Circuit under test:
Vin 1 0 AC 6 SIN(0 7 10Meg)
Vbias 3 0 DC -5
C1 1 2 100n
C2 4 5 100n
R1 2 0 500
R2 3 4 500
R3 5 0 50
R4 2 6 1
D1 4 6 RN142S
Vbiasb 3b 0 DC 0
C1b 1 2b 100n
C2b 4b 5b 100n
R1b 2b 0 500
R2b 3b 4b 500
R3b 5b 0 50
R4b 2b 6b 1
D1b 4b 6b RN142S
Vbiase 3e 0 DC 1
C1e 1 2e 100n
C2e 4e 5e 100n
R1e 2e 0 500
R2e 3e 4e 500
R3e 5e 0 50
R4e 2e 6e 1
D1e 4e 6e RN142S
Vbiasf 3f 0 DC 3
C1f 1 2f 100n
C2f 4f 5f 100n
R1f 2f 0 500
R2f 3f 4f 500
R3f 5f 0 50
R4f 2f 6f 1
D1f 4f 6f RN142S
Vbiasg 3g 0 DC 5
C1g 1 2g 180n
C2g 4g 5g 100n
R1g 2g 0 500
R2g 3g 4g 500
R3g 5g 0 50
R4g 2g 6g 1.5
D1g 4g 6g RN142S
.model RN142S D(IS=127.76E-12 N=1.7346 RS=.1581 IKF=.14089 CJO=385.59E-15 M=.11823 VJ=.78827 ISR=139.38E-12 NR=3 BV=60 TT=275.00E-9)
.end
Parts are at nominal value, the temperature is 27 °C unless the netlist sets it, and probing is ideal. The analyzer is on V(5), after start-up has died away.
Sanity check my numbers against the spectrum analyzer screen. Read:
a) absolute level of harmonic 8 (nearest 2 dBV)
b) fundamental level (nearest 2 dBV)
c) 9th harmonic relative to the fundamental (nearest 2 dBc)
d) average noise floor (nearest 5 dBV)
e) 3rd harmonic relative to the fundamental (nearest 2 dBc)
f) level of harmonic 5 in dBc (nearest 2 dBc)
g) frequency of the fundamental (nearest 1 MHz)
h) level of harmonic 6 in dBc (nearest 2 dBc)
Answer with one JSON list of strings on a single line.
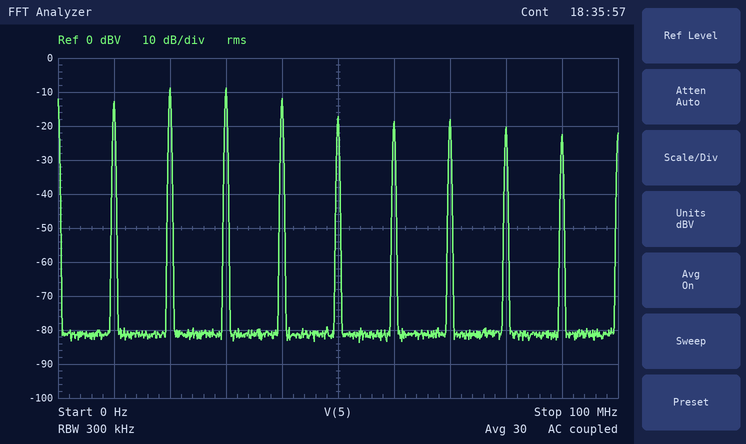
["-20 dBV", "-12 dBV", "-10 dBc", "-80 dBV", "4 dBc", "-4 dBc", "10 MHz", "-6 dBc"]
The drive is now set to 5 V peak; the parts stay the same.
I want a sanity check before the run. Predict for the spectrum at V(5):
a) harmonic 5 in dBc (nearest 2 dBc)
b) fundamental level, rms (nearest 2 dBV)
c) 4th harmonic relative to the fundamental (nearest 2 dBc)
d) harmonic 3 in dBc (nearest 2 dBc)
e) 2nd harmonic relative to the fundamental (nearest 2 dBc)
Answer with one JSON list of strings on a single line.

["-50 dBc", "-50 dBV", "-42 dBc", "-34 dBc", "-24 dBc"]
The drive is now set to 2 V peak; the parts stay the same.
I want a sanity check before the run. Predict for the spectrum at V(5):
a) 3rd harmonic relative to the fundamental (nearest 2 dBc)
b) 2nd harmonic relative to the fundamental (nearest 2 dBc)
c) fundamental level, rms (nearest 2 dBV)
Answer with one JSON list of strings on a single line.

["-54 dBc", "-34 dBc", "-58 dBV"]
